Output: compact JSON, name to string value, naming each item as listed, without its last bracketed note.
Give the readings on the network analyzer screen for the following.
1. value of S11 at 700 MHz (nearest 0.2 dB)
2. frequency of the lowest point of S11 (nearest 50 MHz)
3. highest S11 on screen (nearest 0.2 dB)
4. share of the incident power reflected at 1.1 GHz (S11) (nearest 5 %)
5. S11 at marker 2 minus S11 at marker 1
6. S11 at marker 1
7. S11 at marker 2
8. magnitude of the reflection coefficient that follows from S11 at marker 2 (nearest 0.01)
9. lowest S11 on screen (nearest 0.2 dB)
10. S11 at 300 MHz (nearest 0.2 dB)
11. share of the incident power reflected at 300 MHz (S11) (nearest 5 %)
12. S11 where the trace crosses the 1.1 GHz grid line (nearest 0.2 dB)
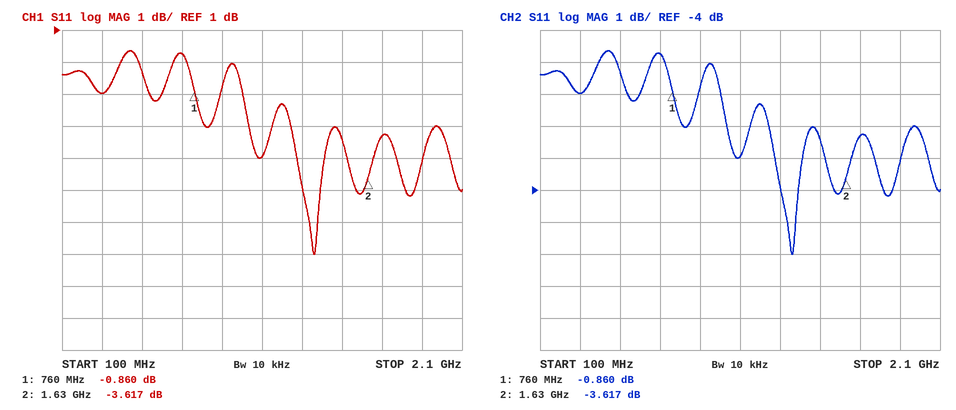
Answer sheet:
{"value of S11 at 700 MHz": "0.2 dB", "frequency of the lowest point of S11": "1.35 GHz", "highest S11 on screen": "0.4 dB", "share of the incident power reflected at 1.1 GHz (S11)": "50 %", "S11 at marker 2 minus S11 at marker 1": "-2.757 dB", "S11 at marker 1": "-0.860 dB", "S11 at marker 2": "-3.617 dB", "magnitude of the reflection coefficient that follows from S11 at marker 2": "0.66", "lowest S11 on screen": "-6.0 dB", "S11 at 300 MHz": "-1.0 dB", "share of the incident power reflected at 300 MHz (S11)": "80 %", "S11 where the trace crosses the 1.1 GHz grid line": "-3.0 dB"}
